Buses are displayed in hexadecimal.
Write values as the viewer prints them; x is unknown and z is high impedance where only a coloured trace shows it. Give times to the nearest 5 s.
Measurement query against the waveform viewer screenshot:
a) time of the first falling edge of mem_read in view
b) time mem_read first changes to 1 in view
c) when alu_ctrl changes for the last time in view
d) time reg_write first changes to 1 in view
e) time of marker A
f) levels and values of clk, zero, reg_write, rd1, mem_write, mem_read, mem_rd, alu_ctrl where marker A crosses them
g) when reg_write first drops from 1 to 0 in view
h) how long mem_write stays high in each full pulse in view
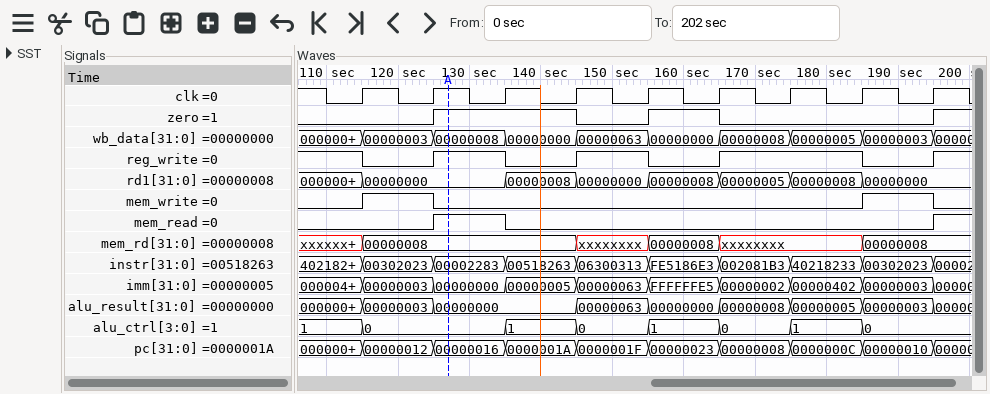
135 s
125 s
185 s
125 s
125 s
clk=1, zero=1, reg_write=1, rd1=00000000, mem_write=0, mem_read=1, mem_rd=00000008, alu_ctrl=0
115 s
10 s, 10 s
